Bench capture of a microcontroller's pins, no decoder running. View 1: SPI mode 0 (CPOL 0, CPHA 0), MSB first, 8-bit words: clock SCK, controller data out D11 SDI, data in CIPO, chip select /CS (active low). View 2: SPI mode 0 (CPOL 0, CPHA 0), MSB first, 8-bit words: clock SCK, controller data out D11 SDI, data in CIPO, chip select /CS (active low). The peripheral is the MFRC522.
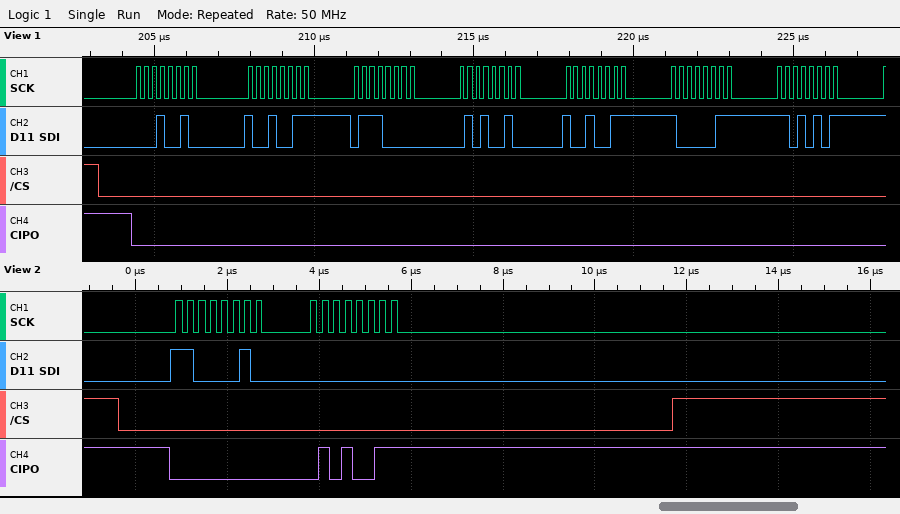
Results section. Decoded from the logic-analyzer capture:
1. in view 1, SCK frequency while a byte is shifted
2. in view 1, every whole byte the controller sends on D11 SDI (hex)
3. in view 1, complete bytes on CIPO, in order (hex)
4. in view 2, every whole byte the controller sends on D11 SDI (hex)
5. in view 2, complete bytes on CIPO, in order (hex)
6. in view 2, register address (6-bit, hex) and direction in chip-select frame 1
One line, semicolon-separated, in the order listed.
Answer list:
4 MHz; 12 93 70 52 93 83 D5; 00 00 00 00 00 00 00; C2 00; 00 53; 0x21 read
